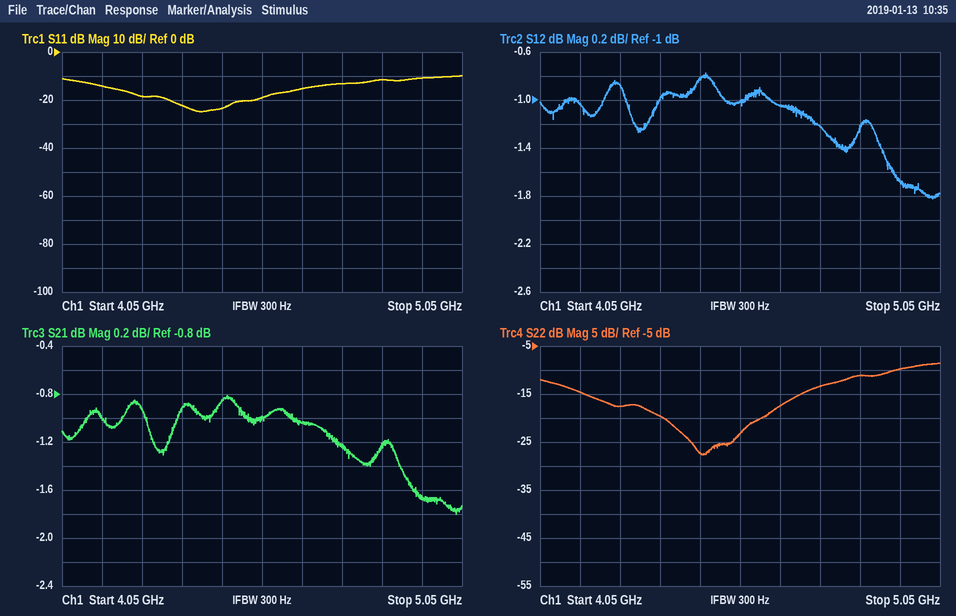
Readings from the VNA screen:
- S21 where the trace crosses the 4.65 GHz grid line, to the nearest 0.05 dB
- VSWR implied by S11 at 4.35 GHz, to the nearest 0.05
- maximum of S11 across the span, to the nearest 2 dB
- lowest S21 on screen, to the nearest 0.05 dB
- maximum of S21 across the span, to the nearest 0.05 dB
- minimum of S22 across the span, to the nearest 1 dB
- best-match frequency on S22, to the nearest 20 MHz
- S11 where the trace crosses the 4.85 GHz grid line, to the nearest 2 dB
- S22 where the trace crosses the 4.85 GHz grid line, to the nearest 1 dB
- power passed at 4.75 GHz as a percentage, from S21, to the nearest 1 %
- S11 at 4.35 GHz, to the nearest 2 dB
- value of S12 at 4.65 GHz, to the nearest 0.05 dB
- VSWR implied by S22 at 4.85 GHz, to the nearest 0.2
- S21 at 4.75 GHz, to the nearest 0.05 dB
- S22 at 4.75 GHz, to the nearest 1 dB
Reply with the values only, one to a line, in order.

-1.05 dB
1.15
-10 dB
-1.80 dB
-0.80 dB
-28 dB
4.46 GHz
-12 dB
-11 dB
75 %
-22 dB
-1.05 dB
1.8
-1.25 dB
-13 dB
